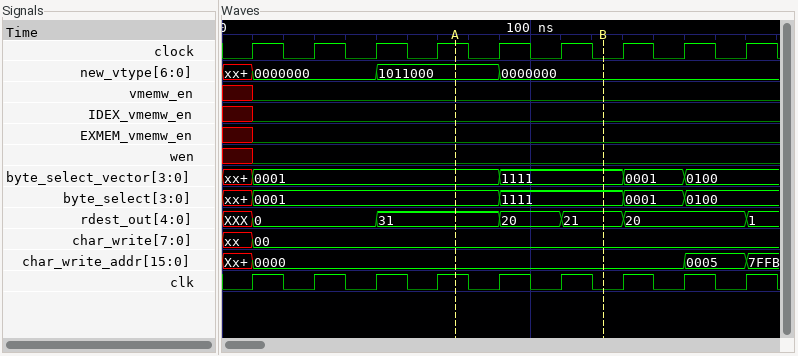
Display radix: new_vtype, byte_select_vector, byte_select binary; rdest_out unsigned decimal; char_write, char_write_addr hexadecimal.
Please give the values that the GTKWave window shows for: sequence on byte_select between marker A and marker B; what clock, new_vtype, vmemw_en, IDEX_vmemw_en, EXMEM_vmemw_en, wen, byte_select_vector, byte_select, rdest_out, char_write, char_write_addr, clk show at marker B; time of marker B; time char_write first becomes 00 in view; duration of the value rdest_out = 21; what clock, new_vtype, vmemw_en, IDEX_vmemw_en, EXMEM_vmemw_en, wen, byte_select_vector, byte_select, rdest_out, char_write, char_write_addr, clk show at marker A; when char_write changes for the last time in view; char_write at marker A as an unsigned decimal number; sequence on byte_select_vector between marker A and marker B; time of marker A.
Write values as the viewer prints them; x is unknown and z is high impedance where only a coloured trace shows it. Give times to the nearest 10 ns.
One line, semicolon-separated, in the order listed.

0001, 1111; clock=0, new_vtype=0000000, vmemw_en=0, IDEX_vmemw_en=0, EXMEM_vmemw_en=0, wen=0, byte_select_vector=1111, byte_select=1111, rdest_out=21, char_write=00, char_write_addr=0000, clk=0; 120 ns; 10 ns; 20 ns; clock=1, new_vtype=1011000, vmemw_en=0, IDEX_vmemw_en=0, EXMEM_vmemw_en=0, wen=0, byte_select_vector=0001, byte_select=0001, rdest_out=31, char_write=00, char_write_addr=0000, clk=1; 10 ns; 0; 0001, 1111; 80 ns
